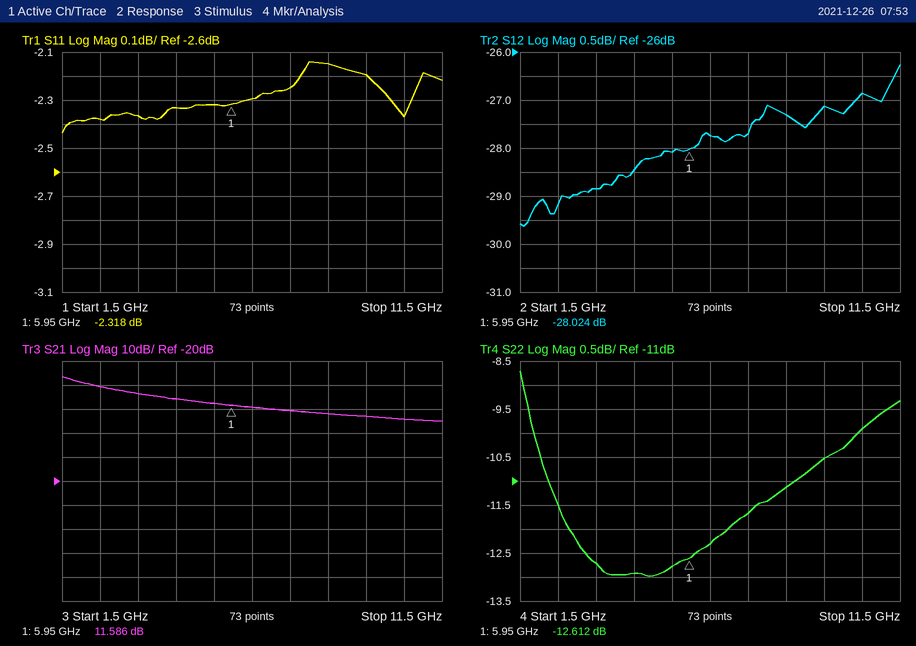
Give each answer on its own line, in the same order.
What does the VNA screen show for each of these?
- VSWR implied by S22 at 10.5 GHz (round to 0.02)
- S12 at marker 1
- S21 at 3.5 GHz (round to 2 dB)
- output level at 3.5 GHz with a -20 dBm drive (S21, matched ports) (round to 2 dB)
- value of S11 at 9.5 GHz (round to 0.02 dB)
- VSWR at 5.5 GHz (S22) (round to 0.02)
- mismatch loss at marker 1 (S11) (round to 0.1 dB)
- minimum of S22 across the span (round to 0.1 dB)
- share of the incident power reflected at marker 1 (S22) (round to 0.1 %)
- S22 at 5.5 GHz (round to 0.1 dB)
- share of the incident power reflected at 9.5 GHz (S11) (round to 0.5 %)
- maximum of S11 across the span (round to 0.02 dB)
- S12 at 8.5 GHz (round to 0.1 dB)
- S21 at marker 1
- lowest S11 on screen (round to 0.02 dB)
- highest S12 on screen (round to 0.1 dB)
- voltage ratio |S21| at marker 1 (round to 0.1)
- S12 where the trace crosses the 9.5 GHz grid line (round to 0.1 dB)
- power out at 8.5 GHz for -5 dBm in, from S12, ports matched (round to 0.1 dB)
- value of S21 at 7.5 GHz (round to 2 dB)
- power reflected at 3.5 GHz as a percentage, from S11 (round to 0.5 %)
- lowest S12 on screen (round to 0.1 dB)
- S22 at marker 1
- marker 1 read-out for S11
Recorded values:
1.94
-28.024 dB
16 dB
-4 dBm
-2.20 dB
1.60
3.8 dB
-13.0 dB
5.5 %
-12.8 dB
60.5 %
-2.14 dB
-27.3 dB
11.586 dB
-2.44 dB
-26.3 dB
3.8
-27.1 dB
-32.3 dBm
10 dB
58.0 %
-29.6 dB
-12.612 dB
-2.318 dB
